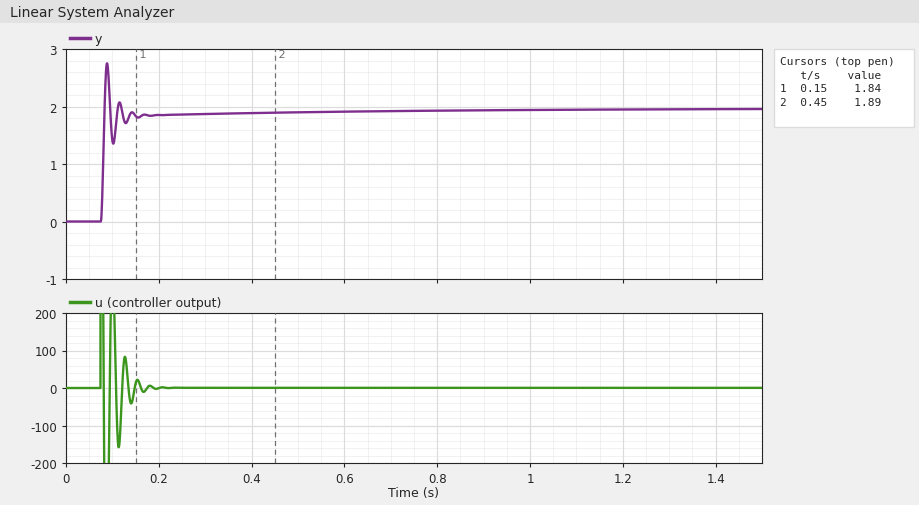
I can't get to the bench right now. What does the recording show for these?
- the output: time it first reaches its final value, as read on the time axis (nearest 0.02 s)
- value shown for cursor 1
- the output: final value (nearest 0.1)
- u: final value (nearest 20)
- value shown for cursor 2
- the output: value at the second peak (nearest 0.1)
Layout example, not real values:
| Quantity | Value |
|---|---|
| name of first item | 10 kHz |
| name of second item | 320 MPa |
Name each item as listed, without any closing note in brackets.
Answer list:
| Quantity | Value |
|---|---|
| the output: time it first reaches its final value, as read on the time axis | 0.08 s |
| value shown for cursor 1 | 1.84 |
| the output: final value | 2.0 |
| u: final value | 0 |
| value shown for cursor 2 | 1.89 |
| the output: value at the second peak | 2.1 |
